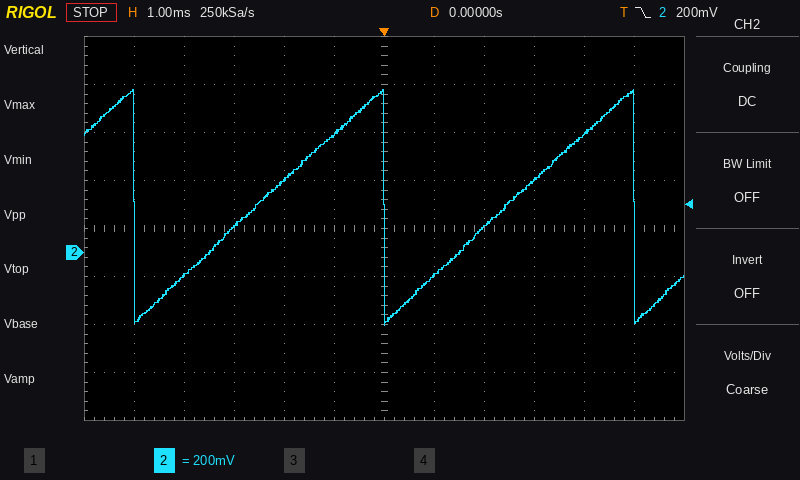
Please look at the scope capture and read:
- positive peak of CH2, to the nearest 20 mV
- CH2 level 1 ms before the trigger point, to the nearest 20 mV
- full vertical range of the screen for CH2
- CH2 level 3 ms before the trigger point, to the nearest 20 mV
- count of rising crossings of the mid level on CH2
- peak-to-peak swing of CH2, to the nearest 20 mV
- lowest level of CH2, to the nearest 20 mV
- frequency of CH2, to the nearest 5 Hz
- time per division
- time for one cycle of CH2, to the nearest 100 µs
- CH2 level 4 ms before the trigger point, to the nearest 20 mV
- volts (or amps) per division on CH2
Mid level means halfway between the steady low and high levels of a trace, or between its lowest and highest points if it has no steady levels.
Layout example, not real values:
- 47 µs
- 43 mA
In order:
- 680 mV
- 500 mV
- 1.6 V
- 120 mV
- 2
- 980 mV
- -300 mV
- 200 Hz
- 1 ms
- 5.0 ms
- -100 mV
- 200 mV
